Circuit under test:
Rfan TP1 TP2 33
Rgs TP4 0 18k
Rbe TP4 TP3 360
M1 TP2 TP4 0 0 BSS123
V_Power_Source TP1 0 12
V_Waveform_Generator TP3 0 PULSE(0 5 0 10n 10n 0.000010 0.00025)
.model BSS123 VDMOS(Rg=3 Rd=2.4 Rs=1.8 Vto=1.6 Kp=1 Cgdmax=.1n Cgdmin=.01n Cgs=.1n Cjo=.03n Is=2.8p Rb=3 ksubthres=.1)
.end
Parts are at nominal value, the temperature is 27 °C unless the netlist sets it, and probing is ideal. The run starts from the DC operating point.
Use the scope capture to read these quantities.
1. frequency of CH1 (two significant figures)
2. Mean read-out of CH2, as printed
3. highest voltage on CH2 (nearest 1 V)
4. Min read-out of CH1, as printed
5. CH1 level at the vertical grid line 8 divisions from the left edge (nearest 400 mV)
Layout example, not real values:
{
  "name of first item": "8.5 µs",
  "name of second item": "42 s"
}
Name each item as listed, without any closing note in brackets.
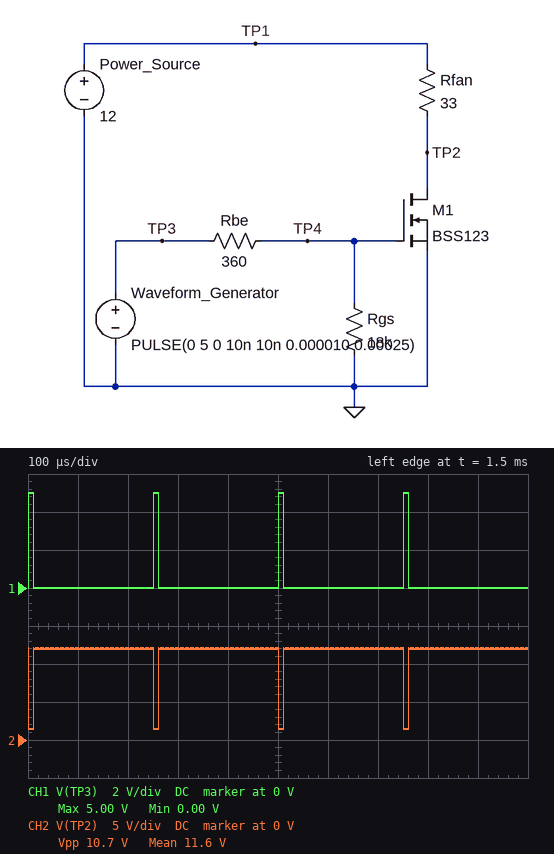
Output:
{
  "frequency of CH1": "4.0 kHz",
  "Mean read-out of CH2, as printed": "11.6 V",
  "highest voltage on CH2": "12 V",
  "Min read-out of CH1, as printed": "0.00 V",
  "CH1 level at the vertical grid line 8 divisions from the left edge": "0 V"
}
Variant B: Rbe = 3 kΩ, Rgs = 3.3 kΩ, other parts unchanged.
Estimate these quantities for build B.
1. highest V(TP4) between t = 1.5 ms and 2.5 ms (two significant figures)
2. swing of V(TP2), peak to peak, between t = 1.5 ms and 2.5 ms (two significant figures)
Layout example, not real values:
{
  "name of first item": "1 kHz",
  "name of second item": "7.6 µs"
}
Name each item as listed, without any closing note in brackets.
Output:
{
  "highest V(TP4) between t = 1.5 ms and 2.5 ms": "2.6 V",
  "swing of V(TP2), peak to peak, between t = 1.5 ms and 2.5 ms": "6.9 V"
}
